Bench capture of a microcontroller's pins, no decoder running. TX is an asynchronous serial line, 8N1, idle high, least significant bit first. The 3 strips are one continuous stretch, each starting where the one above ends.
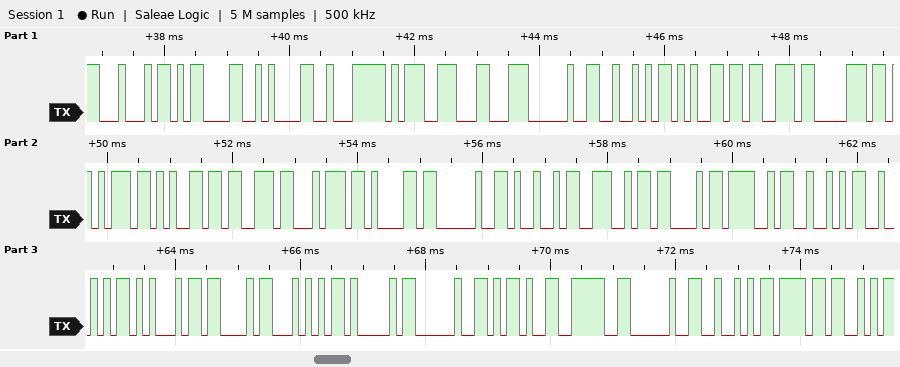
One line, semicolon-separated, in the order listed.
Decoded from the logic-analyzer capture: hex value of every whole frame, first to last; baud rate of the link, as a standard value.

0x44 0x0D 0x0A 0xE2 0x9D 0x8C 0x20 0x52 0x65 0x73 0x70 0x75 0x65 0x73 0x74 0x61 0x20 0x49 0x4E 0x43 0x4F 0x52 0x52 0x45 0x43 0x54 0x41 0x20 0x2D 0x3E 0x20 0x52 0x6F; 9600 baud
